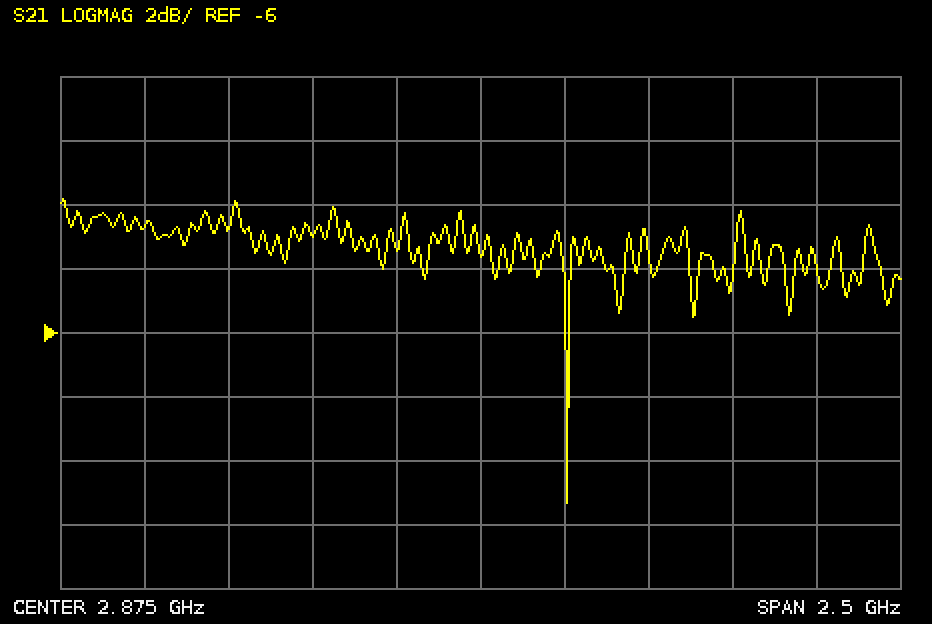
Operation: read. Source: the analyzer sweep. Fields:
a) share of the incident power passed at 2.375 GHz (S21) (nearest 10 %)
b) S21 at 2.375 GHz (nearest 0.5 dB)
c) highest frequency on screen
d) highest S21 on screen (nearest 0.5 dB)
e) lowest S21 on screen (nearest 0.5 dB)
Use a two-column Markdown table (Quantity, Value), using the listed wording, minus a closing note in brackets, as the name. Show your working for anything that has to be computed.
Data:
| Quantity | Value |
|---|---|
| share of the incident power passed at 2.375 GHz (S21) | 10^(-3/10) ≈ 50 % |
| S21 at 2.375 GHz | -3.0 dB |
| highest frequency on screen | 4.125 GHz |
| highest S21 on screen | -2.0 dB |
| lowest S21 on screen | -11.5 dB |
